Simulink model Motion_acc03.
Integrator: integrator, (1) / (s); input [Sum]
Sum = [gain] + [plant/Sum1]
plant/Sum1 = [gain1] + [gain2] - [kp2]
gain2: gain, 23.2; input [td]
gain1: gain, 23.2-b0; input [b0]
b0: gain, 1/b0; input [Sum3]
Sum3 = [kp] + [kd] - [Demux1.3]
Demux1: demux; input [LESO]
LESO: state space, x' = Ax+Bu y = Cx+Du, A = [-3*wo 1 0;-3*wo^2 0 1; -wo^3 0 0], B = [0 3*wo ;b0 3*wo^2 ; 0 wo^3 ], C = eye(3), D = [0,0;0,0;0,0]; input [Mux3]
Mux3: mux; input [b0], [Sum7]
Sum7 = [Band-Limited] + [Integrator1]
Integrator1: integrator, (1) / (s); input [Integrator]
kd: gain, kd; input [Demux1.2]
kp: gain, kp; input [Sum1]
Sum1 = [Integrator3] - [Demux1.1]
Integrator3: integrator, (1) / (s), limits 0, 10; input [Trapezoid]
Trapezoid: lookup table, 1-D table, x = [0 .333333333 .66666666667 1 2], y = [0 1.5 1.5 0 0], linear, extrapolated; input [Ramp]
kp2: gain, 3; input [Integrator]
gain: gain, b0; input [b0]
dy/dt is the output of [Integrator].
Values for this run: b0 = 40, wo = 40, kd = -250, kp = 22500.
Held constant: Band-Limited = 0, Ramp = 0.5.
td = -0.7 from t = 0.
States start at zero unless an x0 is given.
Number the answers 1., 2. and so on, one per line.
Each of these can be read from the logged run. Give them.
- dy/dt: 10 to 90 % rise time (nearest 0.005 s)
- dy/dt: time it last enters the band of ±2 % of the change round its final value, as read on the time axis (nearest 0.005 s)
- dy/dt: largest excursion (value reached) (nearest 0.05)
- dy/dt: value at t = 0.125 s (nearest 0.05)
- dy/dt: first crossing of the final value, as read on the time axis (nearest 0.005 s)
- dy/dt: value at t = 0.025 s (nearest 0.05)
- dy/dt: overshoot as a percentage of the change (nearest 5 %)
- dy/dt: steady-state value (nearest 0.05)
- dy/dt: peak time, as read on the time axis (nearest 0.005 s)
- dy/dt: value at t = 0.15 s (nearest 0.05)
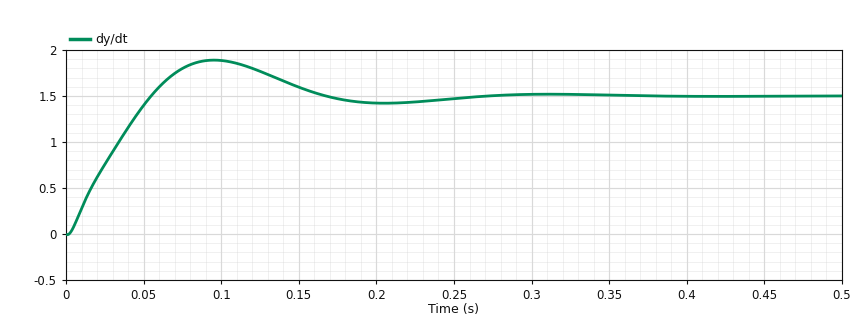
1. 0.040 s
2. 0.250 s
3. 1.90
4. 1.75
5. 0.055 s
6. 0.75
7. 25 %
8. 1.50
9. 0.095 s
10. 1.60
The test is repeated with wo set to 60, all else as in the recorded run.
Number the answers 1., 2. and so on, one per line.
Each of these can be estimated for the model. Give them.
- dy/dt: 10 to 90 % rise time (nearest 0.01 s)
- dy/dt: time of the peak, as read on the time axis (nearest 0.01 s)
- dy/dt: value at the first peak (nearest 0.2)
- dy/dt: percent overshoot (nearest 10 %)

1. 0.03 s
2. 0.07 s
3. 2.0
4. 30 %
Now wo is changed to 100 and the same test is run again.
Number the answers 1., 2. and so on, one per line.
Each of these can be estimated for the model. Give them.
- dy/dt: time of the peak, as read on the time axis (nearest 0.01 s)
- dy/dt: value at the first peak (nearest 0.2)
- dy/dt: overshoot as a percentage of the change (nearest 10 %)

1. 0.05 s
2. 2.0
3. 30 %
